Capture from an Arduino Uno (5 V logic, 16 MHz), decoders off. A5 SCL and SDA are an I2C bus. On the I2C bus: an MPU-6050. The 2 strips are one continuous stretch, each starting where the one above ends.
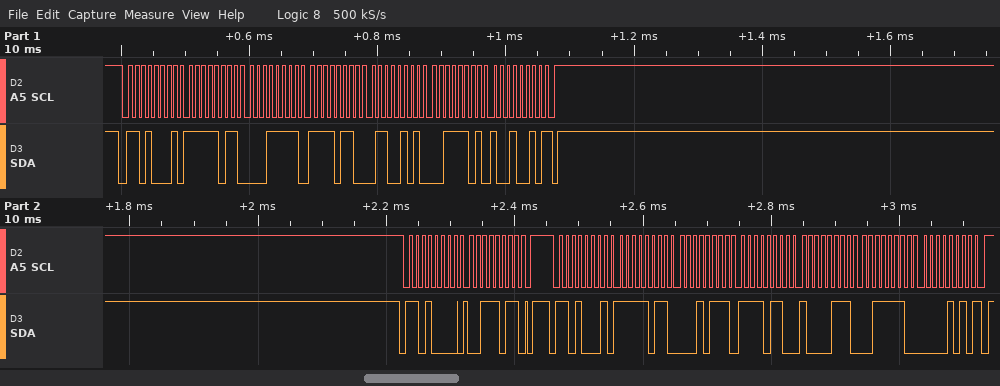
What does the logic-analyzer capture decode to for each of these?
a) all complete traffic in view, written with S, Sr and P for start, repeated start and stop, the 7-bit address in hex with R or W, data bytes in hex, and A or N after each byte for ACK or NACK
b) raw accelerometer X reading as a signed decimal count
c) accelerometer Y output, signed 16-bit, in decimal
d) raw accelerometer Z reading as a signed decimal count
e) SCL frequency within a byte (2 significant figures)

S 68R A FB A 1F A F6 A 65 A 3D A 92 N P S 68W A 3B A P S 68R A FB A 17 A F6 A 87 A 3E A 0A N P
-1257
-2425
15882
100 kHz
